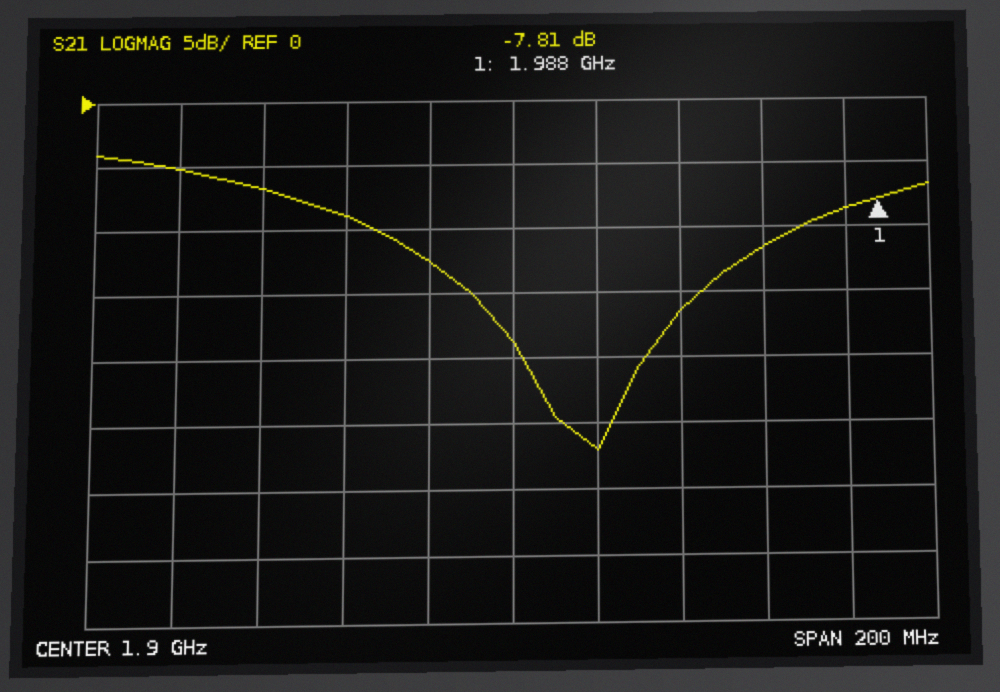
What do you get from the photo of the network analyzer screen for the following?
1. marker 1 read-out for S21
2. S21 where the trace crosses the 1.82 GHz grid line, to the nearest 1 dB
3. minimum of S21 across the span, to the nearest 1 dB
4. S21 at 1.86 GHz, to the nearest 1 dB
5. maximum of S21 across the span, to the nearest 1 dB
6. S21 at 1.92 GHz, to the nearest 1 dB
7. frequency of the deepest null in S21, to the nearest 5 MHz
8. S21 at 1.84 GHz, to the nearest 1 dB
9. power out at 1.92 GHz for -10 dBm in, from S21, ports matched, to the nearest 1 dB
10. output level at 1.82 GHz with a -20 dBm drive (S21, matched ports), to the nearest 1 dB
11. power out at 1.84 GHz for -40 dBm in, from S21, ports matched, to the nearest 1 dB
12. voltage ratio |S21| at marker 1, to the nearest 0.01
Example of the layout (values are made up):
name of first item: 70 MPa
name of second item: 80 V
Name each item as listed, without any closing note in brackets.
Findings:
marker 1 read-out for S21: -7.81 dB
S21 where the trace crosses the 1.82 GHz grid line, to the nearest 1 dB: -5 dB
minimum of S21 across the span, to the nearest 1 dB: -27 dB
S21 at 1.86 GHz, to the nearest 1 dB: -9 dB
maximum of S21 across the span, to the nearest 1 dB: -4 dB
S21 at 1.92 GHz, to the nearest 1 dB: -27 dB
frequency of the deepest null in S21, to the nearest 5 MHz: 1.920 GHz
S21 at 1.84 GHz, to the nearest 1 dB: -7 dB
power out at 1.92 GHz for -10 dBm in, from S21, ports matched, to the nearest 1 dB: -37 dBm
output level at 1.82 GHz with a -20 dBm drive (S21, matched ports), to the nearest 1 dB: -25 dBm
power out at 1.84 GHz for -40 dBm in, from S21, ports matched, to the nearest 1 dB: -47 dBm
voltage ratio |S21| at marker 1, to the nearest 0.01: 0.41
